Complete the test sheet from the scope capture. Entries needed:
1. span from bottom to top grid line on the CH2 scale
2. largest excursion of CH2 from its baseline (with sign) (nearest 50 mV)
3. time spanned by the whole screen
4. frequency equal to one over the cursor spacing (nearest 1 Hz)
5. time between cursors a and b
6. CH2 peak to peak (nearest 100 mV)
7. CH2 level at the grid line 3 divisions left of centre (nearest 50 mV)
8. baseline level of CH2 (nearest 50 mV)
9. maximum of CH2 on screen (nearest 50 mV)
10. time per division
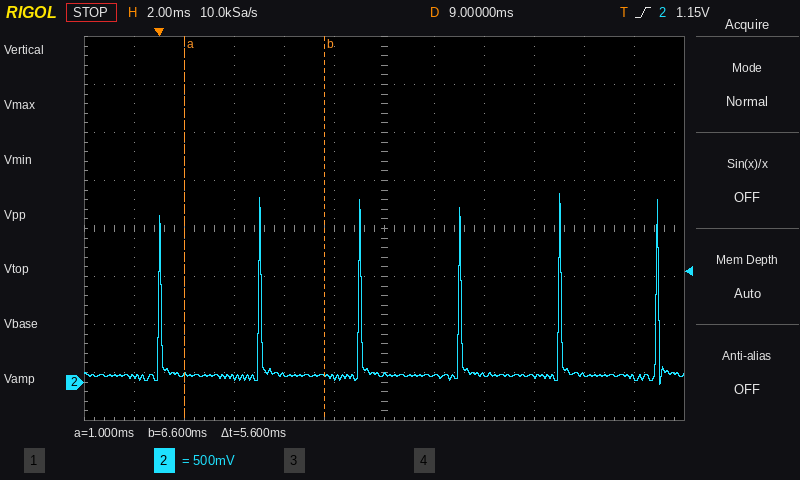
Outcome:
4 V
+1.90 V
24 ms
179 Hz
5.6 ms
2.00 V
50 mV
50 mV
1.95 V
2 ms
